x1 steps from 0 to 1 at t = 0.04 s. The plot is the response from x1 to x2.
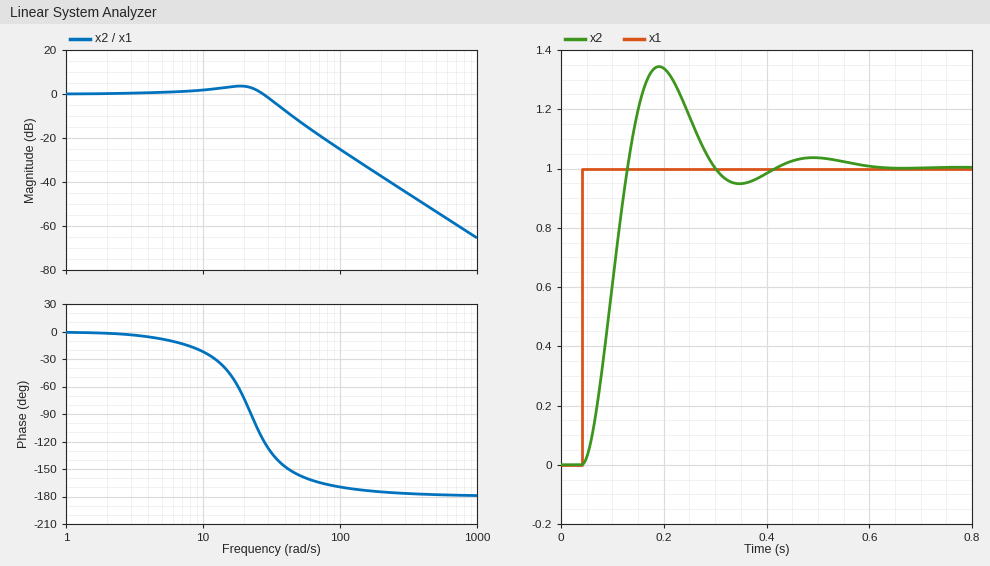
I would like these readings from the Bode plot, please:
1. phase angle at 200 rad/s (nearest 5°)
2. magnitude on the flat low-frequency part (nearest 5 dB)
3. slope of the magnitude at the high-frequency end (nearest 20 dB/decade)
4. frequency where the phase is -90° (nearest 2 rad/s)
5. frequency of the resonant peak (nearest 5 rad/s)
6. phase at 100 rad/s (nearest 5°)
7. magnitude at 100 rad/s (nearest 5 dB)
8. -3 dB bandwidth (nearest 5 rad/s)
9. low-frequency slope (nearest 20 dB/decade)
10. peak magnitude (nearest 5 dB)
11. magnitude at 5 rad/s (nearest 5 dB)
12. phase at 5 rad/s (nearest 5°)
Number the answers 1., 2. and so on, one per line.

1. -175°
2. 0 dB
3. -40 dB/decade
4. 22 rad/s
5. 20 rad/s
6. -170°
7. -25 dB
8. 30 rad/s
9. 0 dB/decade
10. 5 dB
11. 0 dB
12. -10°
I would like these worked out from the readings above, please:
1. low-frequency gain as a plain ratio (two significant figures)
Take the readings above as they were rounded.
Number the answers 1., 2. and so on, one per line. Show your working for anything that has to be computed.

1. 10^(0 / 20) = 1.0
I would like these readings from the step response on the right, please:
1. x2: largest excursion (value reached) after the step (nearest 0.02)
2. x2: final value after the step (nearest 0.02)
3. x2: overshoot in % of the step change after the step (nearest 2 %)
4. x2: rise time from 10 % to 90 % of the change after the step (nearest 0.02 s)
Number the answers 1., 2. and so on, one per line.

1. 1.34
2. 1.00
3. 34 %
4. 0.06 s
